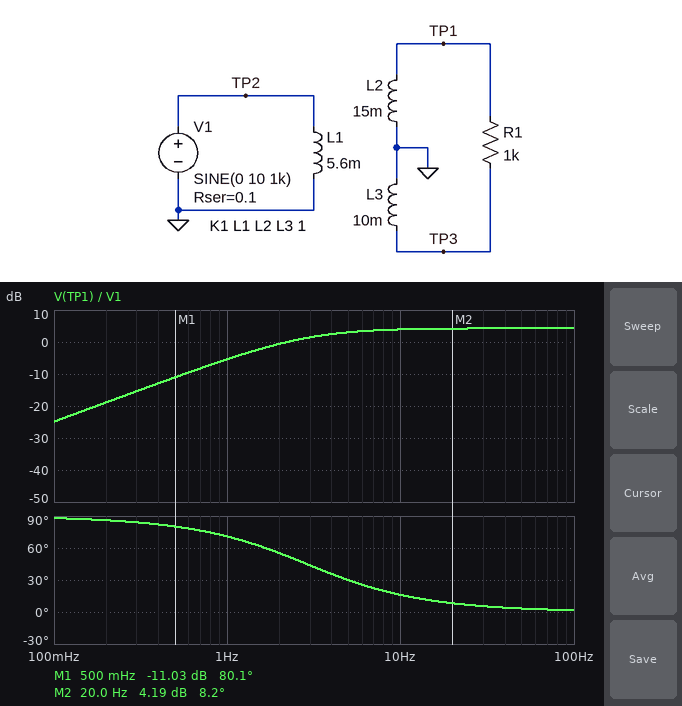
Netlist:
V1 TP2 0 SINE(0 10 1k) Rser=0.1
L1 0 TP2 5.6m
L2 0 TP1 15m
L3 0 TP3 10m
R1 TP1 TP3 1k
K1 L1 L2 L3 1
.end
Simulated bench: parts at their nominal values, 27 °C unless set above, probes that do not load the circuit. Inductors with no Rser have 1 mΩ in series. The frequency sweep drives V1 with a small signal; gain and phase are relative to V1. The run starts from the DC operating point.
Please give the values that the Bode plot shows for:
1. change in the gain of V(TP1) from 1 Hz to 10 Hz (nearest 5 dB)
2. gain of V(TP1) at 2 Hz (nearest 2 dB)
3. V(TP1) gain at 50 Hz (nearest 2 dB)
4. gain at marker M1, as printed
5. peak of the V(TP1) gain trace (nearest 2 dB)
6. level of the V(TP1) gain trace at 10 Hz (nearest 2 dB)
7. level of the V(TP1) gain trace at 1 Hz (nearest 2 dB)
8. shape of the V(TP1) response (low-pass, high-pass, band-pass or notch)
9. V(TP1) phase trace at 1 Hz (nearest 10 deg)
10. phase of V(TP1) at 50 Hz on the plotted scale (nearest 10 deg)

10 dB
0 dB
4 dB
-11.03 dB
4 dB
4 dB
-6 dB
high-pass
70 deg
0 deg
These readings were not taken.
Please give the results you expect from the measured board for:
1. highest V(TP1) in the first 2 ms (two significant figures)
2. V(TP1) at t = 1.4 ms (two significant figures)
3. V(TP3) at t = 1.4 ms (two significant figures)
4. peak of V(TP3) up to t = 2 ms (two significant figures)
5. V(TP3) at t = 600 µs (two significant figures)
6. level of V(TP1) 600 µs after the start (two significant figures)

16 V
9.5 V
7.8 V
13 V
-7.9 V
-9.7 V
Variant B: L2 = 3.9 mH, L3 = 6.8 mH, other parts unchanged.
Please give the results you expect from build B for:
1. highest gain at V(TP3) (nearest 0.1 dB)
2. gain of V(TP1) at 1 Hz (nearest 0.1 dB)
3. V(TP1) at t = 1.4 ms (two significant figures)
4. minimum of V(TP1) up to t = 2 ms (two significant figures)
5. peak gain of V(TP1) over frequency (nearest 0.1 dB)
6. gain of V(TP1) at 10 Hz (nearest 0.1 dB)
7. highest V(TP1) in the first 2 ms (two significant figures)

0.8 dB
-11.2 dB
4.9 V
-8.4 V
-1.6 dB
-1.9 dB
8.3 V
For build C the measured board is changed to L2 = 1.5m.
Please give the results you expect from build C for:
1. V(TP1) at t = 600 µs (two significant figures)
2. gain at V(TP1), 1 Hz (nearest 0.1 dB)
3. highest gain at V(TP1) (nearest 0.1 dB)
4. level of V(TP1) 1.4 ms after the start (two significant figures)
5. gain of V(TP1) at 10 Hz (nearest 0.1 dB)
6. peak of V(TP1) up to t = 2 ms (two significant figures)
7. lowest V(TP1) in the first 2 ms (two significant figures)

-3.1 V
-15.4 dB
-5.7 dB
3.0 V
-6.1 dB
5.2 V
-5.2 V
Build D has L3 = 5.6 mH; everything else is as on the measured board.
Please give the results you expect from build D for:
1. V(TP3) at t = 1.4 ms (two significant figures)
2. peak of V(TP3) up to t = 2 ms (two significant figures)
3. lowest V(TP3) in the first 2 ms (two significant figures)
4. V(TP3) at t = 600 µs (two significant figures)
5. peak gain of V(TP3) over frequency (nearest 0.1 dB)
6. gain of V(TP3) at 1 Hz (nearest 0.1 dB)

5.8 V
10 V
-10 V
-5.9 V
0 dB
-9.7 dB
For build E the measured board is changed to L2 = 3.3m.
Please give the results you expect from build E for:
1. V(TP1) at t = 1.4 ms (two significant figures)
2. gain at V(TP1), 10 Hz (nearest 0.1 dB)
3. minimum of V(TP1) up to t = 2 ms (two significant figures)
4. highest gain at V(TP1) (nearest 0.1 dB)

4.5 V
-2.6 dB
-7.7 V
-2.3 dB
